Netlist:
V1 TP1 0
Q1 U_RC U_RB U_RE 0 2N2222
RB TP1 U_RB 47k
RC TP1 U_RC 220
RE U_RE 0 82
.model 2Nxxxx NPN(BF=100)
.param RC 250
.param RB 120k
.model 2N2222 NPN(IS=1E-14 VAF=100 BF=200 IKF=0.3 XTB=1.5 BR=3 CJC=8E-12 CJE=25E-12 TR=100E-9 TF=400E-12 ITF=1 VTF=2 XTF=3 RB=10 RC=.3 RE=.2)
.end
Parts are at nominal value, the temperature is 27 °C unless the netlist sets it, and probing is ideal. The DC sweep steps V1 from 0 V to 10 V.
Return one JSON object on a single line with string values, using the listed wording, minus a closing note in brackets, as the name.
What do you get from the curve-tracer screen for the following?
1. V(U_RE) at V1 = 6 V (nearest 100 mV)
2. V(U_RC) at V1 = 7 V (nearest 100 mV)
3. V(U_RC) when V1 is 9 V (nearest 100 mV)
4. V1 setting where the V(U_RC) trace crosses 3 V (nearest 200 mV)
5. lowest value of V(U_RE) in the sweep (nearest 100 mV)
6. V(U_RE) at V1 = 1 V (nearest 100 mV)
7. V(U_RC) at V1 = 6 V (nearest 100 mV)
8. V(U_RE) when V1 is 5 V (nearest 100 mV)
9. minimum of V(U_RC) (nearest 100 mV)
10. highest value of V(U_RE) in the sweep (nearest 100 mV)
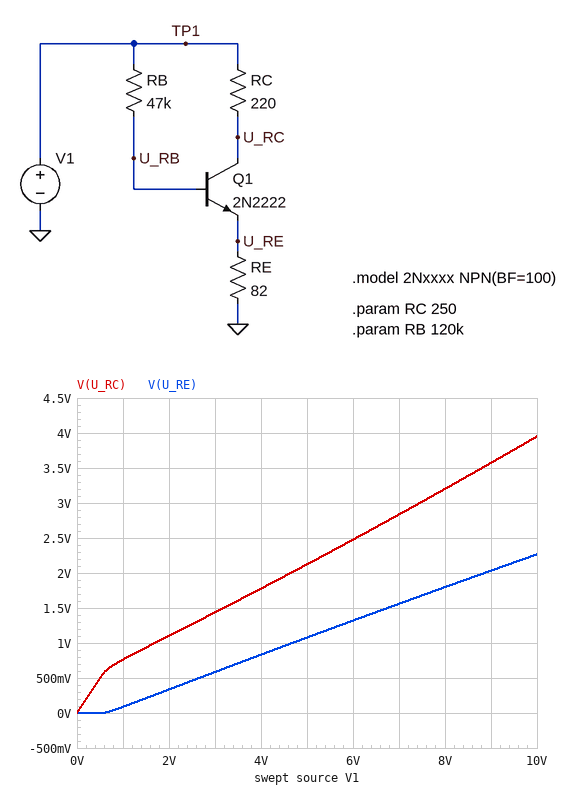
{"V(U_RE) at V1 = 6 V": "1.3 V", "V(U_RC) at V1 = 7 V": "2.8 V", "V(U_RC) when V1 is 9 V": "3.6 V", "V1 setting where the V(U_RC) trace crosses 3 V": "7.4 V", "lowest value of V(U_RE) in the sweep": "0 V", "V(U_RE) at V1 = 1 V": "100 mV", "V(U_RC) at V1 = 6 V": "2.5 V", "V(U_RE) when V1 is 5 V": "1.1 V", "minimum of V(U_RC)": "0 V", "highest value of V(U_RE) in the sweep": "2.3 V"}
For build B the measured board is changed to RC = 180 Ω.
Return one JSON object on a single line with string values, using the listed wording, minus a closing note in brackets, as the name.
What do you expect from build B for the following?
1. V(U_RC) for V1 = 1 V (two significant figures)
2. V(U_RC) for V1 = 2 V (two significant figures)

{"V(U_RC) for V1 = 1 V": "810 mV", "V(U_RC) for V1 = 2 V": "1.3 V"}
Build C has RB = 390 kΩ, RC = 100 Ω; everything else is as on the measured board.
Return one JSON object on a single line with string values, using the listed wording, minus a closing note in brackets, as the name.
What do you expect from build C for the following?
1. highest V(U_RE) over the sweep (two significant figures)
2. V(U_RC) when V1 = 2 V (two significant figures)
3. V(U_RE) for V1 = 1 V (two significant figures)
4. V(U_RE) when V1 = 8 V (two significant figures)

{"highest V(U_RE) over the sweep": "400 mV", "V(U_RC) when V1 = 2 V": "1.9 V", "V(U_RE) for V1 = 1 V": "16 mV", "V(U_RE) when V1 = 8 V": "310 mV"}
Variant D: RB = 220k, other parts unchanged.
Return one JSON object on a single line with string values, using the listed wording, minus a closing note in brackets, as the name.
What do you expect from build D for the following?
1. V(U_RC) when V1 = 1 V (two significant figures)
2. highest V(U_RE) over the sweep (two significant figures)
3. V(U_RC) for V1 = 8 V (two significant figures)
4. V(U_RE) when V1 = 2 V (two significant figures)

{"V(U_RC) when V1 = 1 V": "930 mV", "highest V(U_RE) over the sweep": "670 mV", "V(U_RC) for V1 = 8 V": "6.6 V", "V(U_RE) when V1 = 2 V": "94 mV"}
